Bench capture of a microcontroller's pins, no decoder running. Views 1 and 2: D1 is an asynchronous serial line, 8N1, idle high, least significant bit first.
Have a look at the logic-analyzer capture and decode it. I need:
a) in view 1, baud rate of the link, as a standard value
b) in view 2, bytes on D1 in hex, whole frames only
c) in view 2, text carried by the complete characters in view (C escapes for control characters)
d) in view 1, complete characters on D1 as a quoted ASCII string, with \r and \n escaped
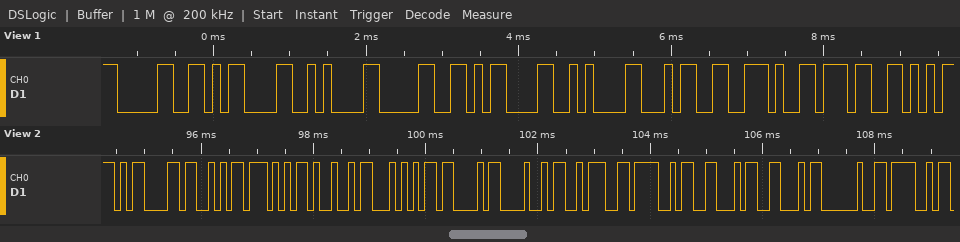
9600 baud
0D 53 57 49 54 43 48 3A 4F 46 46 20 4F
"\rSWITCH:OFF O"
"0\r\n0\r\n4.7"
